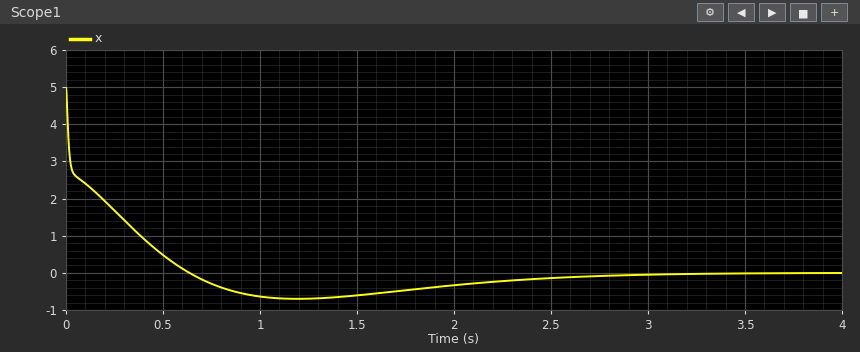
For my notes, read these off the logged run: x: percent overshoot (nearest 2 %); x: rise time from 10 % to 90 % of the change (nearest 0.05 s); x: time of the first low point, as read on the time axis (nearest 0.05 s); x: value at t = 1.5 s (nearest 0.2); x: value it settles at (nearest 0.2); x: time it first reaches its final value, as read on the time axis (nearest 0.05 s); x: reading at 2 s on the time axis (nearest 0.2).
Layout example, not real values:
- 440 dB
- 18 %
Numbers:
- 14 %
- 0.50 s
- 1.20 s
- -0.6
- 0.0
- 0.65 s
- -0.4
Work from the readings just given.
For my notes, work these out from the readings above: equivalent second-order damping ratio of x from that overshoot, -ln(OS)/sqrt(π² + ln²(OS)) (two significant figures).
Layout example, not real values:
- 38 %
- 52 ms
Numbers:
- 0.53
